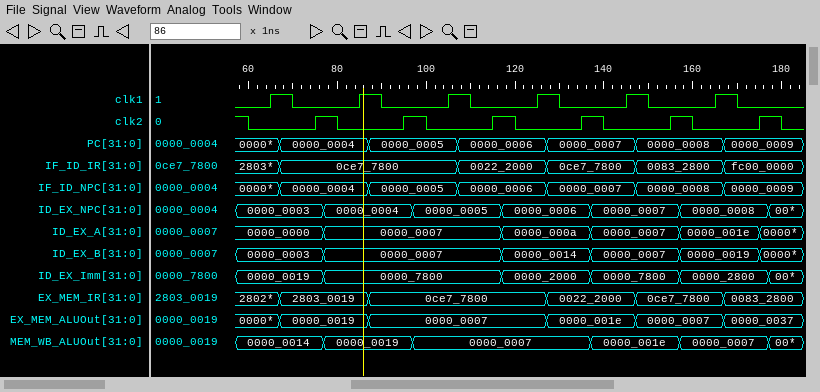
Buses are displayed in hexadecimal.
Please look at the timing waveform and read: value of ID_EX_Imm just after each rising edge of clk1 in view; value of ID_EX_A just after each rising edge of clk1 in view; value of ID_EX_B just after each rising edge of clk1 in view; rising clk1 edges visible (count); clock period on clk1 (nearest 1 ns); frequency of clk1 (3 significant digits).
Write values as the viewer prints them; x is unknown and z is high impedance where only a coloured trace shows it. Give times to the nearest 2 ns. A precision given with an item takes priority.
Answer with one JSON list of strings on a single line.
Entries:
["0000_0019, 0000_7800, 0000_7800, 0000_2000, 0000_7800, 0000_2800", "0000_0000, 0000_0007, 0000_0007, 0000_000a, 0000_0007, 0000_001e", "0000_0003, 0000_0007, 0000_0007, 0000_0014, 0000_0007, 0000_0019", "6", "20 ns", "50.0 MHz"]
